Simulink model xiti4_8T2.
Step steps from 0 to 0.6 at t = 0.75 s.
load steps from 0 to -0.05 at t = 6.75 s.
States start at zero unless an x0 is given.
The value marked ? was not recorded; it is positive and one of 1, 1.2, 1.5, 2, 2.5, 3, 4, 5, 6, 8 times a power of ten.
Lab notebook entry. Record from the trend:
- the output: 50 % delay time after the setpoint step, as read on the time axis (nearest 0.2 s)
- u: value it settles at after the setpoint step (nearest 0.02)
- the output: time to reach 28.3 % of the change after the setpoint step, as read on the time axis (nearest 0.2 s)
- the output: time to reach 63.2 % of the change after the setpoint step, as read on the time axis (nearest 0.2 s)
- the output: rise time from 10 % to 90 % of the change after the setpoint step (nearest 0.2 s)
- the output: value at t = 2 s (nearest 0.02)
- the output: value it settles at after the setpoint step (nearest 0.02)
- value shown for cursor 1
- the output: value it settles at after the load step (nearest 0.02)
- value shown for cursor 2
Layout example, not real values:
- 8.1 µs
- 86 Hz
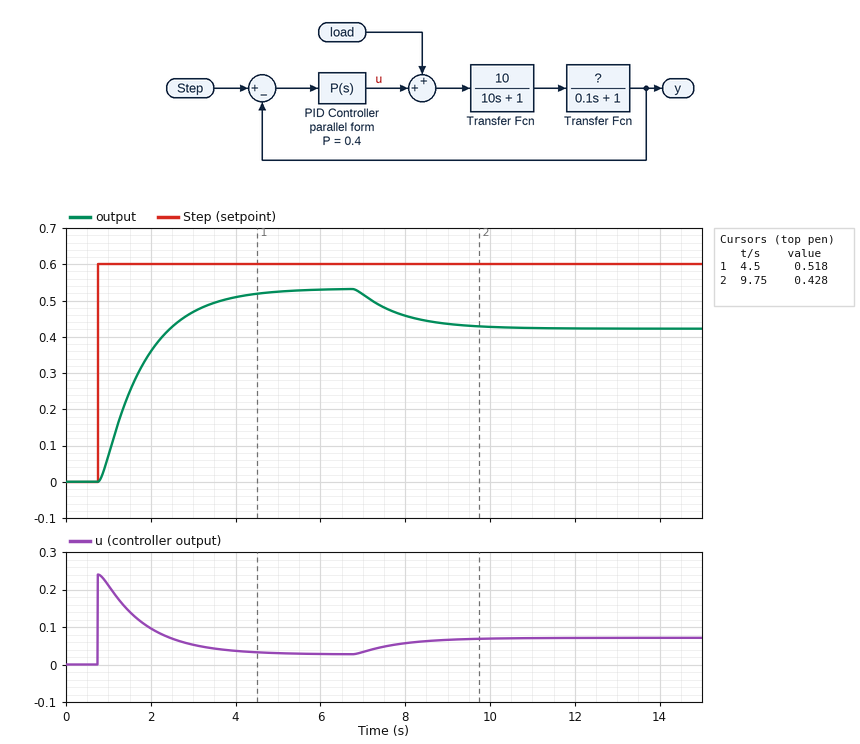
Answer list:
- 1.6 s
- 0.02
- 1.2 s
- 1.8 s
- 2.2 s
- 0.36
- 0.54
- 0.518
- 0.42
- 0.428
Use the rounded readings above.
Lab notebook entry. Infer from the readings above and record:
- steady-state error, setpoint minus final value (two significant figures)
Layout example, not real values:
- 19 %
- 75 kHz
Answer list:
- 0.060
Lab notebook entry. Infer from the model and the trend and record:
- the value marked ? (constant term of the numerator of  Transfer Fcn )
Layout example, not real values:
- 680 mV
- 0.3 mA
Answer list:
- 2
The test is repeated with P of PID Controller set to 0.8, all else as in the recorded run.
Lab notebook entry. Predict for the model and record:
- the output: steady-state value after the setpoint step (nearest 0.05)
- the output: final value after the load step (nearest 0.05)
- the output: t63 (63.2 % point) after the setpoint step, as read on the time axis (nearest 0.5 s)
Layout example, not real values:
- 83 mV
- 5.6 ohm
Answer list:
- 0.55
- 0.50
- 1.5 s
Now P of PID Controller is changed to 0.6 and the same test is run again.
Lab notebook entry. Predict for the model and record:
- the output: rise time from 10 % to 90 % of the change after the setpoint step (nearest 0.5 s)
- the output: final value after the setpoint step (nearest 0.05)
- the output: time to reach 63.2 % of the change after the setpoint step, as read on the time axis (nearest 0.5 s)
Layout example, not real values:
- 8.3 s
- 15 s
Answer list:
- 1.5 s
- 0.55
- 1.5 s
